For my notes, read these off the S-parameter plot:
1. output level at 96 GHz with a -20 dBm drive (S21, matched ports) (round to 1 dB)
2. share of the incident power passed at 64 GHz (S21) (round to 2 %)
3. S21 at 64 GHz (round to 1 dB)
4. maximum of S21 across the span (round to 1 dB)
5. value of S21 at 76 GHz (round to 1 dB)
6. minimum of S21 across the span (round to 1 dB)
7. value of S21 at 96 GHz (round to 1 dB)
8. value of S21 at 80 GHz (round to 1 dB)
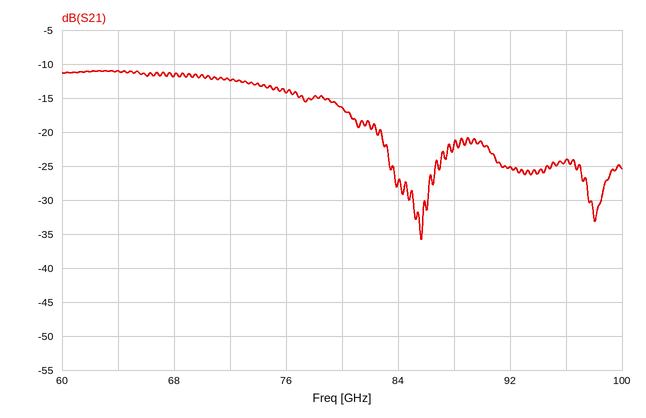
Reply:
-44 dBm
8 %
-11 dB
-11 dB
-14 dB
-36 dB
-24 dB
-16 dB
